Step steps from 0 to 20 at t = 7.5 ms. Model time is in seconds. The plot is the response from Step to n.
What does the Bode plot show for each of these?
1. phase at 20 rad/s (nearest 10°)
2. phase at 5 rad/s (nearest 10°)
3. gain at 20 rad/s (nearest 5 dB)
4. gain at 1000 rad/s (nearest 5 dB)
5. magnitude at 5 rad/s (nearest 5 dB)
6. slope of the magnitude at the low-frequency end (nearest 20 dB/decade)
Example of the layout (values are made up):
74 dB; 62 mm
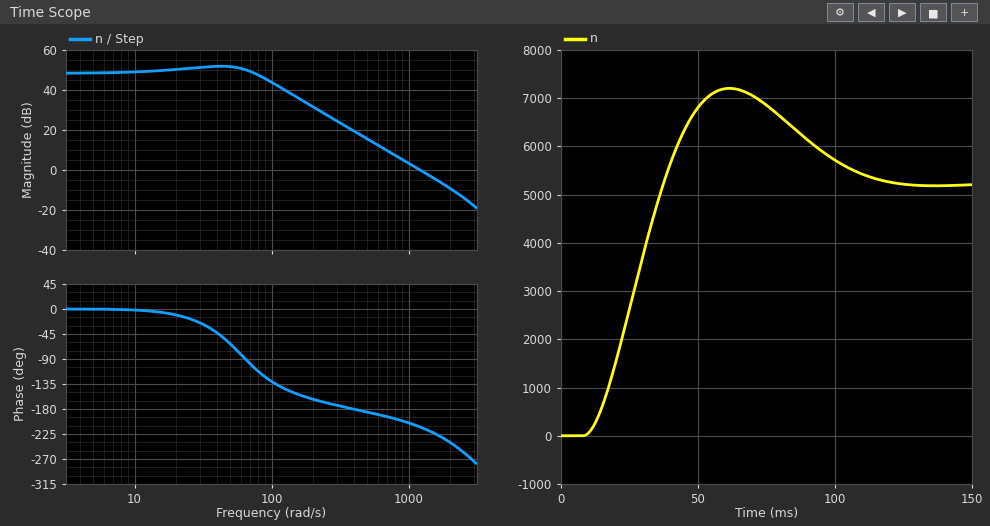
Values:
-10°; 0°; 50 dB; 5 dB; 50 dB; 0 dB/decade
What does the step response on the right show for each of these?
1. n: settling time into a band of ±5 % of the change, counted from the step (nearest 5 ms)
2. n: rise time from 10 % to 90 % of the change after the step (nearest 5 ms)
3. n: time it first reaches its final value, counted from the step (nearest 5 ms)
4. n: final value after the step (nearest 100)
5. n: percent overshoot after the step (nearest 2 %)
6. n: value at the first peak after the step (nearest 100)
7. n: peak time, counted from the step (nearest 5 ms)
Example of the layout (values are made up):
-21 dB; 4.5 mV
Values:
100 ms; 20 ms; 30 ms; 5200; 38 %; 7200; 55 ms
